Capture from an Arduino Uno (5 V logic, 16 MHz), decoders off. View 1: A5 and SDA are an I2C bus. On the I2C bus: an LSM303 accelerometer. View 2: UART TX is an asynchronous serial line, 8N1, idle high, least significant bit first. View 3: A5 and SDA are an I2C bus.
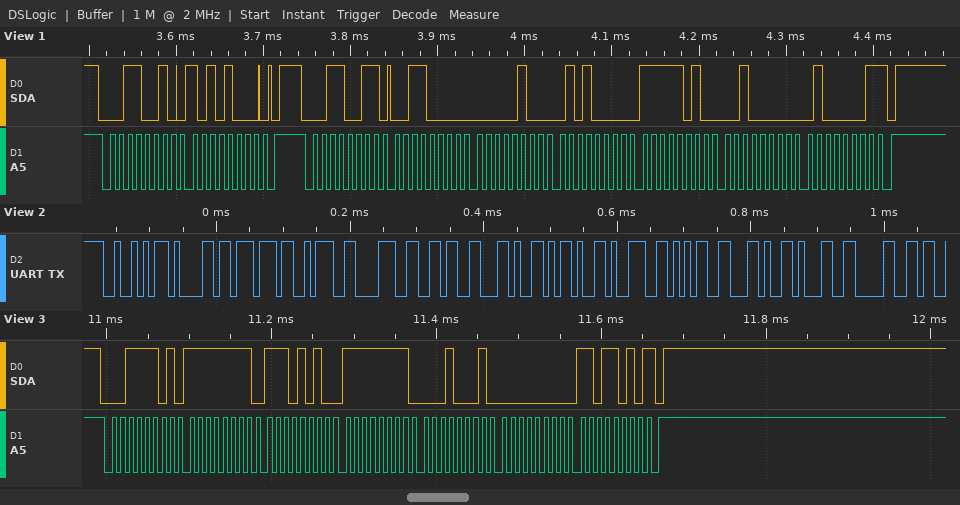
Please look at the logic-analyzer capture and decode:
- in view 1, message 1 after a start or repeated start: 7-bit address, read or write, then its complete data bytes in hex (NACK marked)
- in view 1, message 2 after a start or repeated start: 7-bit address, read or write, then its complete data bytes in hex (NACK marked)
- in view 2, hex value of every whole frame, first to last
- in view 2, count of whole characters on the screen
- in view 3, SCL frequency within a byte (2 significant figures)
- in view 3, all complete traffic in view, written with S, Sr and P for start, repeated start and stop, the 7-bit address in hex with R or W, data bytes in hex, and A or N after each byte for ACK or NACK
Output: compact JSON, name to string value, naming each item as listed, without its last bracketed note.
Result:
{"in view 1, message 1 after a start or repeated start: 7-bit address, read or write, then its complete data bytes in hex": "0x19 write: A8", "in view 1, message 2 after a start or repeated start: 7-bit address, read or write, then its complete data bytes in hex": "0x19 read: 30 04 50 FA 20 41 NACK", "in view 2, hex value of every whole frame, first to last": "52 61 77 3A 38 36 2C 2D 39 35 2C 31 30", "in view 2, count of whole characters on the screen": "13", "in view 3, SCL frequency within a byte": "100 kHz", "in view 3, all complete traffic in view, written with S, Sr and P for start, repeated start and stop, the 7-bit address in hex with R or W, data bytes in hex, and A or N after each byte for ACK or NACK": "S 1ER A FF A EA A FF A 11 A 00 A DA N P"}
